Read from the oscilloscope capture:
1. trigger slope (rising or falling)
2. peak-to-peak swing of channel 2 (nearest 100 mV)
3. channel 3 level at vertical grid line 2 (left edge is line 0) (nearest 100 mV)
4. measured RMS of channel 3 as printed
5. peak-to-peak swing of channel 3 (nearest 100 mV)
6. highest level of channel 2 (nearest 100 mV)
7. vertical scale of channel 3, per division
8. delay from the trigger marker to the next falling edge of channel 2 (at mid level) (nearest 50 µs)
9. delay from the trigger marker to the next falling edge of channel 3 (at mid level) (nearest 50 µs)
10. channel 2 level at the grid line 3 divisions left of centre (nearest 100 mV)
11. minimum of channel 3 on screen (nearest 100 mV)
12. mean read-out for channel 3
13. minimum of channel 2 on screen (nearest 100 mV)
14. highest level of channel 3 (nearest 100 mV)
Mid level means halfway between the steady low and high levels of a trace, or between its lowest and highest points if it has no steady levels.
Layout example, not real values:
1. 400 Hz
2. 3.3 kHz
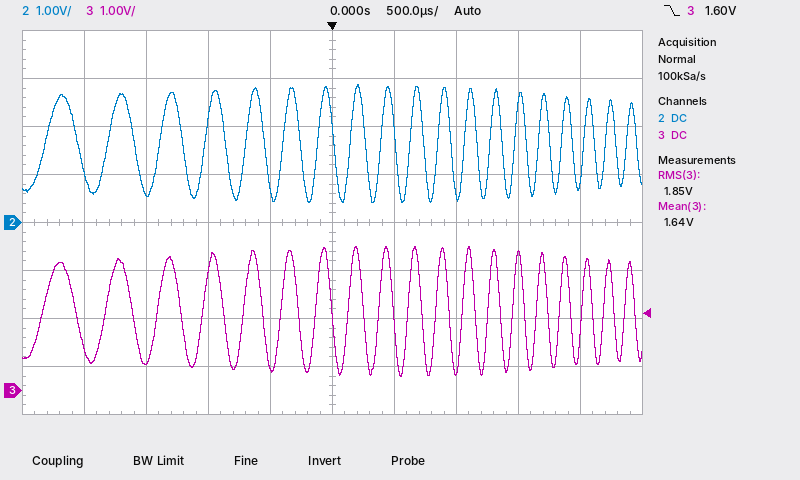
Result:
1. falling
2. 2.5 V
3. 600 mV
4. 1.85 V
5. 2.7 V
6. 2.9 V
7. 1 V
8. 250 µs
9. 250 µs
10. 600 mV
11. 300 mV
12. 1.64 V
13. 400 mV
14. 3.0 V
